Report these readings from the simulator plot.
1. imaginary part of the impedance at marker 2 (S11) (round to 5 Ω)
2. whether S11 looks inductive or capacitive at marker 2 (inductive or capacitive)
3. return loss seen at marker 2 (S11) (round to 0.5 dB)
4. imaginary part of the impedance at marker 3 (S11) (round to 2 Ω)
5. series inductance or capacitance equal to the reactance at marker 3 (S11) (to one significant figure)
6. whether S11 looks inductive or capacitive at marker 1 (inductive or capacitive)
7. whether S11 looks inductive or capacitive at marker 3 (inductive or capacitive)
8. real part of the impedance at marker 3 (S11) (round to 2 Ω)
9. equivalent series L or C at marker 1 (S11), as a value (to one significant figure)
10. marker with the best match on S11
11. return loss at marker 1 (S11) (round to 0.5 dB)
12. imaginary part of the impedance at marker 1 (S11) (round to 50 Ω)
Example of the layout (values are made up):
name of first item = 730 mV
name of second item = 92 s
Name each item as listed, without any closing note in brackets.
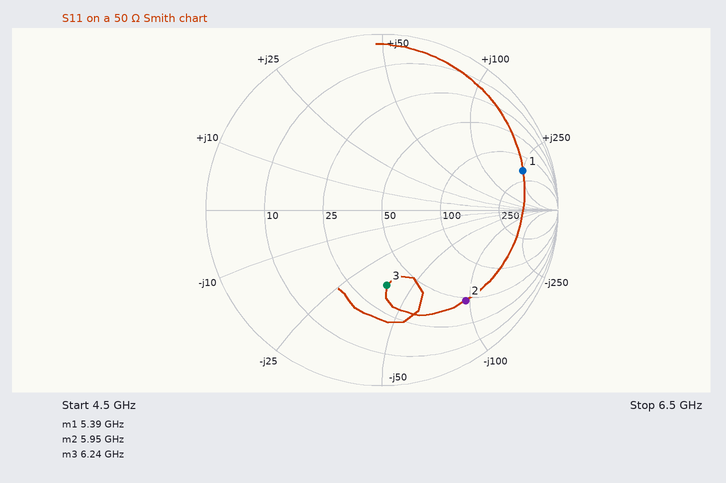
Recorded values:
imaginary part of the impedance at marker 2 (S11) = -95 Ω
whether S11 looks inductive or capacitive at marker 2 = capacitive
return loss seen at marker 2 (S11) = 3.0 dB
imaginary part of the impedance at marker 3 (S11) = -38 Ω
series inductance or capacitance equal to the reactance at marker 3 (S11) = 700 fF
whether S11 looks inductive or capacitive at marker 1 = inductive
whether S11 looks inductive or capacitive at marker 3 = capacitive
real part of the impedance at marker 3 (S11) = 36 Ω
equivalent series L or C at marker 1 (S11), as a value = 7 nH
marker with the best match on S11 = marker 3
return loss at marker 1 (S11) = 1.5 dB
imaginary part of the impedance at marker 1 (S11) = +250 Ω
